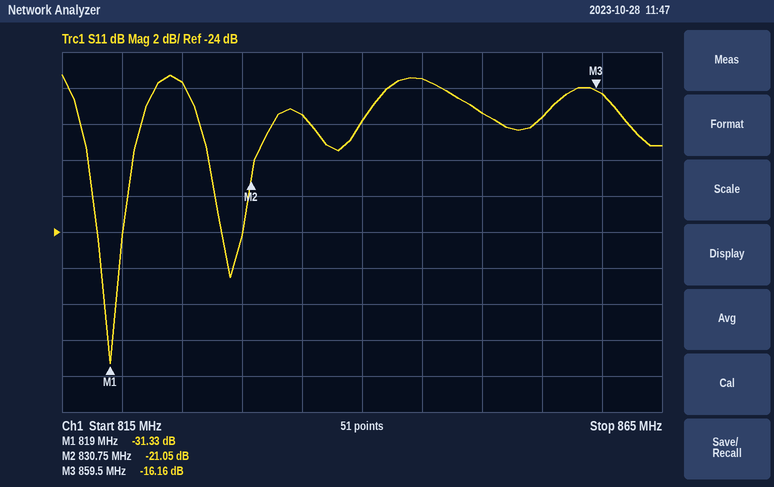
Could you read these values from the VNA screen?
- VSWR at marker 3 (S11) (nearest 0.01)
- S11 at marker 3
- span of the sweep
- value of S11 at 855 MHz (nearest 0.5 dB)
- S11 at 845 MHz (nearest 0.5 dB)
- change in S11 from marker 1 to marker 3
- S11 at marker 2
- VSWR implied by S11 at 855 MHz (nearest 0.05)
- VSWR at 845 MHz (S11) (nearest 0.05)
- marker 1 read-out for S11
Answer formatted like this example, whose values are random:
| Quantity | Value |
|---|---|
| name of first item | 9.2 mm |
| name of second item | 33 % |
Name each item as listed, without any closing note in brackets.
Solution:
| Quantity | Value |
|---|---|
| VSWR at marker 3 (S11) | 1.37 |
| S11 at marker 3 | -16.16 dB |
| span of the sweep | 50 MHz |
| value of S11 at 855 MHz | -17.5 dB |
| S11 at 845 MHz | -15.5 dB |
| change in S11 from marker 1 to marker 3 | 15.17 dB |
| S11 at marker 2 | -21.05 dB |
| VSWR implied by S11 at 855 MHz | 1.30 |
| VSWR at 845 MHz (S11) | 1.40 |
| marker 1 read-out for S11 | -31.33 dB |
